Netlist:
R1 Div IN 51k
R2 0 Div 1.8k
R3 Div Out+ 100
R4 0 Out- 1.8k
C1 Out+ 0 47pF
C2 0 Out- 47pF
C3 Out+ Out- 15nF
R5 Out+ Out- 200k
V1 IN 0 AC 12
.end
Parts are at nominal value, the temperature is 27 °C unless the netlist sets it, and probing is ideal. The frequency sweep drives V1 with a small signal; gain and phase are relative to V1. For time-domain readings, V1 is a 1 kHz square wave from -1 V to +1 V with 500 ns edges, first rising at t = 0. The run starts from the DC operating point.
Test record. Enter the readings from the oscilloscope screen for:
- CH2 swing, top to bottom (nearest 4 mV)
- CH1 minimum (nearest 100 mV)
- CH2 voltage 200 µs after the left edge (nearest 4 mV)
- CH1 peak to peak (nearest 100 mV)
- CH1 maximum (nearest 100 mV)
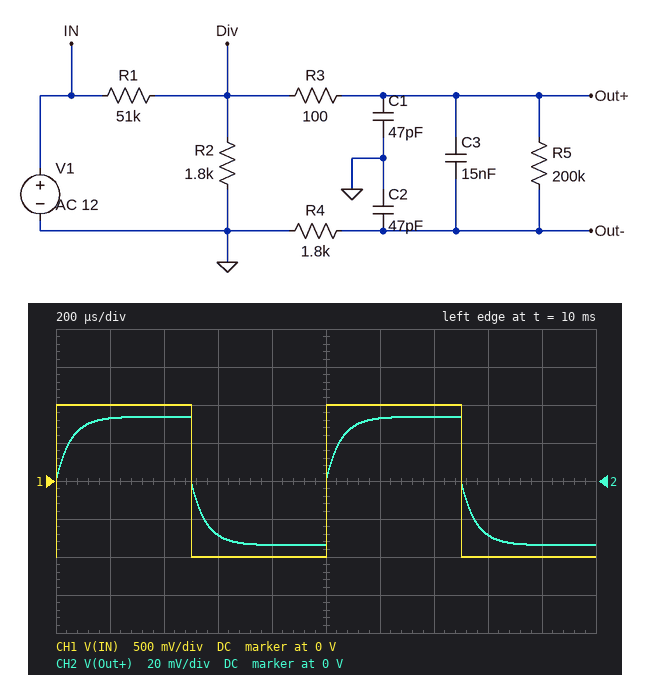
68 mV
-1.0 V
32 mV
2.0 V
1.0 V
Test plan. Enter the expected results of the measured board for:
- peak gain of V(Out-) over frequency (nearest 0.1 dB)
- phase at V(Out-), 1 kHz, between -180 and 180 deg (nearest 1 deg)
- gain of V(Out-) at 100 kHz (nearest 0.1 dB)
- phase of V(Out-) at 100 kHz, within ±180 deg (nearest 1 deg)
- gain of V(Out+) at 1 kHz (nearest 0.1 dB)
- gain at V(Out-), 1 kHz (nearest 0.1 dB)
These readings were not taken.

-35.5 dB
68 deg
-35.5 dB
-1 deg
-29.8 dB
-45.4 dB
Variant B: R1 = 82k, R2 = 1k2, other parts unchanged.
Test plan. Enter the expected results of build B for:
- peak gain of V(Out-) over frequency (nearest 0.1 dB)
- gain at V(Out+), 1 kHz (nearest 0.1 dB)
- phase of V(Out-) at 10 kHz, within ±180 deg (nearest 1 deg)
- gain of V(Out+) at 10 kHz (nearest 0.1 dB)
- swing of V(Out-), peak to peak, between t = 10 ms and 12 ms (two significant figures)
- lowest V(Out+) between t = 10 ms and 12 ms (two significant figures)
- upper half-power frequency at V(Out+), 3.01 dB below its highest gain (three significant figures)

-41.5 dB
-37.1 dB
19 deg
-40.7 dB
33 mV
-14 mV
6.29 kHz
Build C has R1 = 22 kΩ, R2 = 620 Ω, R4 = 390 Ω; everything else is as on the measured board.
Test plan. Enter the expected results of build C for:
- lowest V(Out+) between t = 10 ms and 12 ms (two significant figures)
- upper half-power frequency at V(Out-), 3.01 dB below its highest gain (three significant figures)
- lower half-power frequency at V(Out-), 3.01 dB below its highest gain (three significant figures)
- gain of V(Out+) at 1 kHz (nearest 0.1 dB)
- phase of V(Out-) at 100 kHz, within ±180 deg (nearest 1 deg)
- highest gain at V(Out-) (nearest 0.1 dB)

-27 mV
6.77 MHz
9.72 kHz
-31.3 dB
5 deg
-40.2 dB
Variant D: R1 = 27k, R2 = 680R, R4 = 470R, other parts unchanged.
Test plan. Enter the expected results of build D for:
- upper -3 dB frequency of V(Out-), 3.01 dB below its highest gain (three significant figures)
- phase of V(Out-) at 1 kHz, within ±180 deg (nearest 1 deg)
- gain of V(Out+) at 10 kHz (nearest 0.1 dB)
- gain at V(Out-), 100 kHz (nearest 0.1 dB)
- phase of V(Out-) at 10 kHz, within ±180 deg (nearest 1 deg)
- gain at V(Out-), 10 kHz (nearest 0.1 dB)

5.84 MHz
80 deg
-35.1 dB
-40.6 dB
40 deg
-43.0 dB
